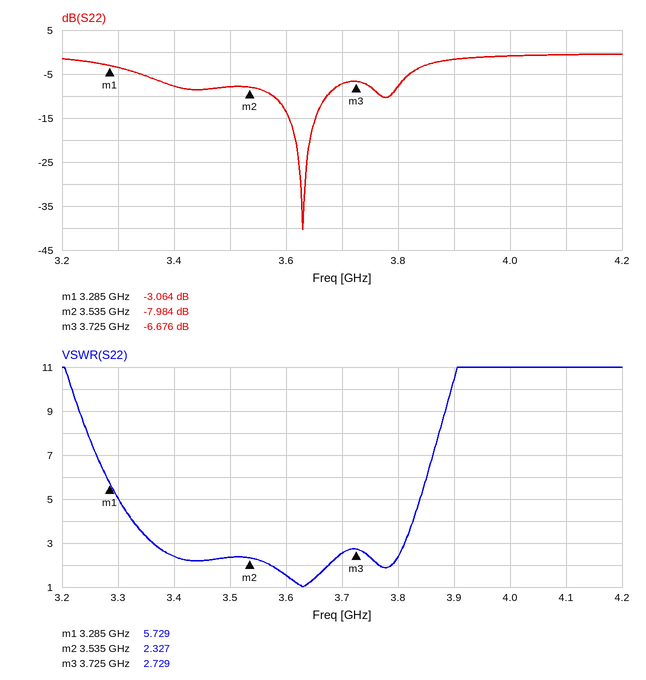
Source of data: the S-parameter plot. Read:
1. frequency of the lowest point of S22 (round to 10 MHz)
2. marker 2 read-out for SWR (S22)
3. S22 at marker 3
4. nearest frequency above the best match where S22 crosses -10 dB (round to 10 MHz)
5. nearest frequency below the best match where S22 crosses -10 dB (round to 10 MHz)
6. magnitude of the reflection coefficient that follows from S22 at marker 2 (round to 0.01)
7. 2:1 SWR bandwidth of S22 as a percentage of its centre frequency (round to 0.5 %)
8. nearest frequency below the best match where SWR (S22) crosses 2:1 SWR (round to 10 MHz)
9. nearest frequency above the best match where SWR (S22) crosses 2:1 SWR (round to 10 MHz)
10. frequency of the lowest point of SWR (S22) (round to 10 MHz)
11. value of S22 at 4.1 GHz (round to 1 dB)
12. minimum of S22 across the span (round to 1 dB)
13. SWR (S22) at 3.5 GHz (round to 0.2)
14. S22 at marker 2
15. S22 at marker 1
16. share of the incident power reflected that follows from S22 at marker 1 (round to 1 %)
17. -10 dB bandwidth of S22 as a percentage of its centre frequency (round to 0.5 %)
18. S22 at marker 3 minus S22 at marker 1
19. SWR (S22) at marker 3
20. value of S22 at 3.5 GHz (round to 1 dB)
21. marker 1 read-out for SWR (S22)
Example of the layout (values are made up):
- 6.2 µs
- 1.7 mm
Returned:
- 3.63 GHz
- 2.327
- -6.676 dB
- 3.67 GHz
- 3.58 GHz
- 0.40
- 3.0 %
- 3.57 GHz
- 3.68 GHz
- 3.63 GHz
- -1 dB
- -40 dB
- 2.4
- -7.984 dB
- -3.064 dB
- 49 %
- 2.5 %
- -3.612 dB
- 2.729
- -8 dB
- 5.729
